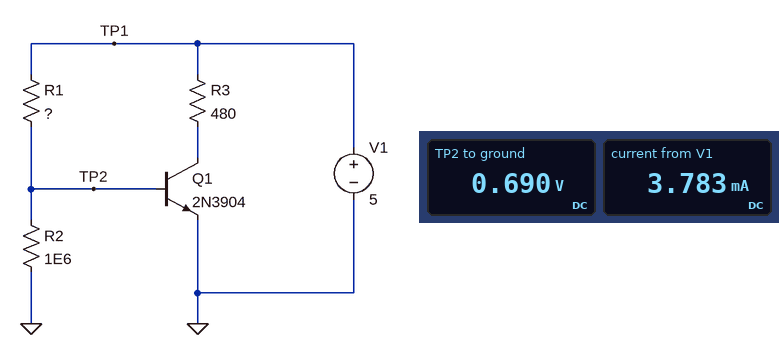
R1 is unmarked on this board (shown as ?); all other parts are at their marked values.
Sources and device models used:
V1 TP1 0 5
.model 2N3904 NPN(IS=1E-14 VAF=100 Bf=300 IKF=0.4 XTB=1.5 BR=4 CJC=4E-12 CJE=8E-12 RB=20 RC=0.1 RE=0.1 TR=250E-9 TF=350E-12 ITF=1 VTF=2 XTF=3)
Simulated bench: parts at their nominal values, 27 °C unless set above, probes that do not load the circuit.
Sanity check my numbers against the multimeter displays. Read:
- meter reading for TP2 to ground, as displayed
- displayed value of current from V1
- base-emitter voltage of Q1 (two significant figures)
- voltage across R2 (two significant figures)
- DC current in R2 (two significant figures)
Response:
0.690 V
3.783 mA
690 mV
690 mV
690 nA
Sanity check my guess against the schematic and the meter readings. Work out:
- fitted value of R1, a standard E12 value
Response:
330 kΩ
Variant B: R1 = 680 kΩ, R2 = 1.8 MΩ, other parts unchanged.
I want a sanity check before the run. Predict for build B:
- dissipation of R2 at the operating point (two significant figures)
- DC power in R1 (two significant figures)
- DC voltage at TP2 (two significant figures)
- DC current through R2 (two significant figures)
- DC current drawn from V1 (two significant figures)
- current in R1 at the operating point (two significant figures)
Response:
250 nW
28 µW
670 mV
370 nA
1.9 mA
6.4 µA
